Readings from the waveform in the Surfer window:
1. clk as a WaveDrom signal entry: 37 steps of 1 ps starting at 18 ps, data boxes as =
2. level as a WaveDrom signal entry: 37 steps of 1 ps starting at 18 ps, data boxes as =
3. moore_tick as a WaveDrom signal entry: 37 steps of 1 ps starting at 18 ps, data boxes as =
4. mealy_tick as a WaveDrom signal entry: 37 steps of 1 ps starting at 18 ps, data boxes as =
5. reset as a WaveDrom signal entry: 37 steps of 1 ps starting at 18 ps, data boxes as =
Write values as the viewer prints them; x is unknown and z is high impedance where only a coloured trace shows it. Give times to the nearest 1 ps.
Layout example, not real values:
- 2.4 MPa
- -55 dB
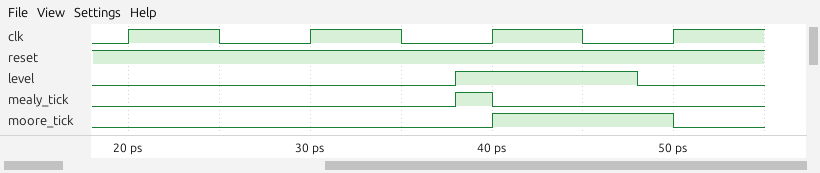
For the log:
- {name: 'clk', wave: '0.1....0....1....0....1....0....1....'}
- {name: 'level', wave: '0...................1.........0......'}
- {name: 'moore_tick', wave: '0.....................1.........0....'}
- {name: 'mealy_tick', wave: '0...................1.0..............'}
- {name: 'reset', wave: '1....................................'}
